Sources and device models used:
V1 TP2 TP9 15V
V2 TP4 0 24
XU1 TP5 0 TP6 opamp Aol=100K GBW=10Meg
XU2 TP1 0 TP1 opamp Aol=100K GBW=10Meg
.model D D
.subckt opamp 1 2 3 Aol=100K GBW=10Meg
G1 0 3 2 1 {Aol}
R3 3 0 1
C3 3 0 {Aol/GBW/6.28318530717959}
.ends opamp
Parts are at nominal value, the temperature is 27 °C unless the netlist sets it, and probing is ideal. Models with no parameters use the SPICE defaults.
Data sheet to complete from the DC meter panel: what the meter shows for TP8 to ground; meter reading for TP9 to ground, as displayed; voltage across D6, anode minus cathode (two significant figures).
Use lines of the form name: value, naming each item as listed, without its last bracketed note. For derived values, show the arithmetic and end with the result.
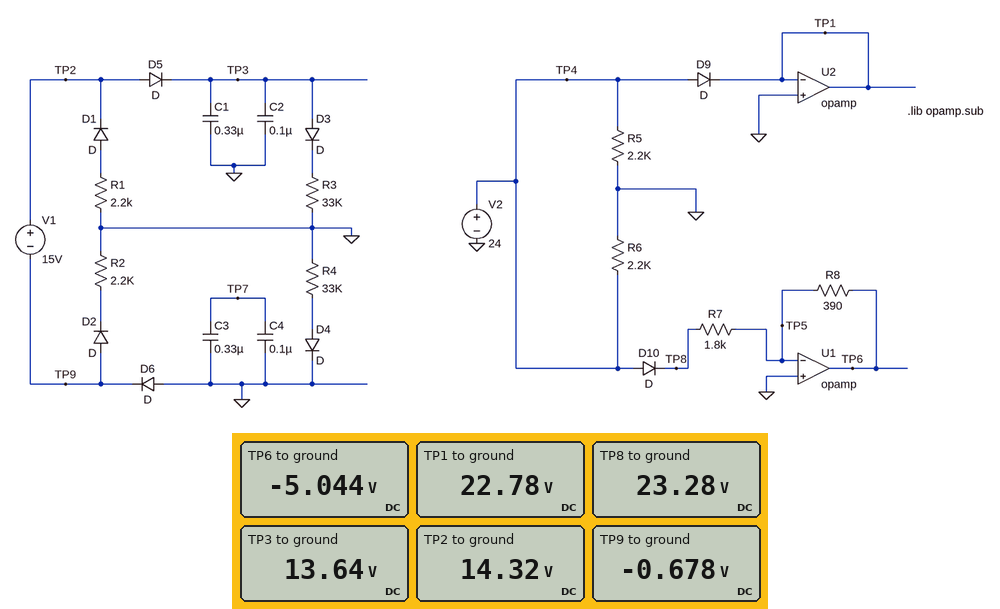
what the meter shows for TP8 to ground: 23.28 V
meter reading for TP9 to ground, as displayed: -0.678 V
voltage across D6, anode minus cathode: 0 V - (-678 mV) = 680 mV
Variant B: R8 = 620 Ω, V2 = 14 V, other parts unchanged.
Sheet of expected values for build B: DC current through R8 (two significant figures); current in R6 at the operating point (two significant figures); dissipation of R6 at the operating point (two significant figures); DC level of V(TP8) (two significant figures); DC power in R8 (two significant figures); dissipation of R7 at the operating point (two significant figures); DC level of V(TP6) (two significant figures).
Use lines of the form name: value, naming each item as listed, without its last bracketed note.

DC current through R8: 7.4 mA
current in R6 at the operating point: 6.4 mA
dissipation of R6 at the operating point: 89 mW
DC level of V(TP8): 13 V
DC power in R8: 34 mW
dissipation of R7 at the operating point: 98 mW
DC level of V(TP6): -4.6 V
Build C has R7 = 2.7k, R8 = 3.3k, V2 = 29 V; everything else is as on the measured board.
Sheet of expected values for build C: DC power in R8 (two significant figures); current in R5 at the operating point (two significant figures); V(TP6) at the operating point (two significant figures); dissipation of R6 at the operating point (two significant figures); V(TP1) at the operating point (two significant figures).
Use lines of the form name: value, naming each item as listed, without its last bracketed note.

DC power in R8: 360 mW
current in R5 at the operating point: 13 mA
V(TP6) at the operating point: -35 V
dissipation of R6 at the operating point: 380 mW
V(TP1) at the operating point: 28 V
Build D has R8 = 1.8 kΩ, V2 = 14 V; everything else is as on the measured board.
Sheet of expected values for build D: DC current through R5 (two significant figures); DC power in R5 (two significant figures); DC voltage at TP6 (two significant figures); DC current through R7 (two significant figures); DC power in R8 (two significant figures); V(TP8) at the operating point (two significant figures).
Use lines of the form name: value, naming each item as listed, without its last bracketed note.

DC current through R5: 6.4 mA
DC power in R5: 89 mW
DC voltage at TP6: -13 V
DC current through R7: 7.4 mA
DC power in R8: 98 mW
V(TP8) at the operating point: 13 V
